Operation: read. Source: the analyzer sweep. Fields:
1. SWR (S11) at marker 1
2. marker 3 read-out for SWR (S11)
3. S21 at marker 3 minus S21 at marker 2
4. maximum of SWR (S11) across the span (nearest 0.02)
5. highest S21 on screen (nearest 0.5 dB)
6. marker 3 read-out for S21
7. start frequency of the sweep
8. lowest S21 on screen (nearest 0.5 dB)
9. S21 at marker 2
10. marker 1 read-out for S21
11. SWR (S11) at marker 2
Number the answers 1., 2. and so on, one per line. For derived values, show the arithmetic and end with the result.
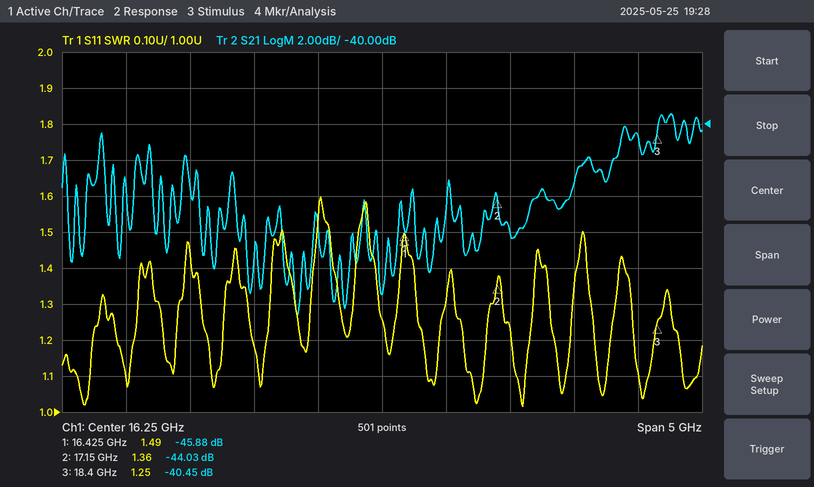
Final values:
1. 1.49
2. 1.25
3. -40.45 − (-44.03) = 3.58 dB
4. 1.60
5. -39.5 dB
6. -40.45 dB
7. 13.75 GHz
8. -50.5 dB
9. -44.03 dB
10. -45.88 dB
11. 1.36
